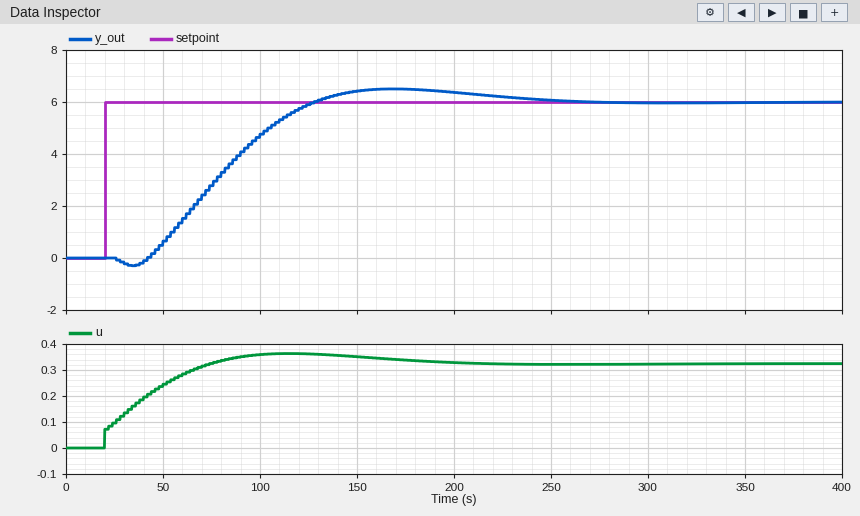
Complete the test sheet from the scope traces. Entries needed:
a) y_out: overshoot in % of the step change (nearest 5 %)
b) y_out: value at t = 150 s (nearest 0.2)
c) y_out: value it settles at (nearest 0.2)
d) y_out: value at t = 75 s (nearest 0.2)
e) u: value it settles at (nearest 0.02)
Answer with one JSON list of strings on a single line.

["10 %", "6.4", "6.0", "2.8", "0.32"]
